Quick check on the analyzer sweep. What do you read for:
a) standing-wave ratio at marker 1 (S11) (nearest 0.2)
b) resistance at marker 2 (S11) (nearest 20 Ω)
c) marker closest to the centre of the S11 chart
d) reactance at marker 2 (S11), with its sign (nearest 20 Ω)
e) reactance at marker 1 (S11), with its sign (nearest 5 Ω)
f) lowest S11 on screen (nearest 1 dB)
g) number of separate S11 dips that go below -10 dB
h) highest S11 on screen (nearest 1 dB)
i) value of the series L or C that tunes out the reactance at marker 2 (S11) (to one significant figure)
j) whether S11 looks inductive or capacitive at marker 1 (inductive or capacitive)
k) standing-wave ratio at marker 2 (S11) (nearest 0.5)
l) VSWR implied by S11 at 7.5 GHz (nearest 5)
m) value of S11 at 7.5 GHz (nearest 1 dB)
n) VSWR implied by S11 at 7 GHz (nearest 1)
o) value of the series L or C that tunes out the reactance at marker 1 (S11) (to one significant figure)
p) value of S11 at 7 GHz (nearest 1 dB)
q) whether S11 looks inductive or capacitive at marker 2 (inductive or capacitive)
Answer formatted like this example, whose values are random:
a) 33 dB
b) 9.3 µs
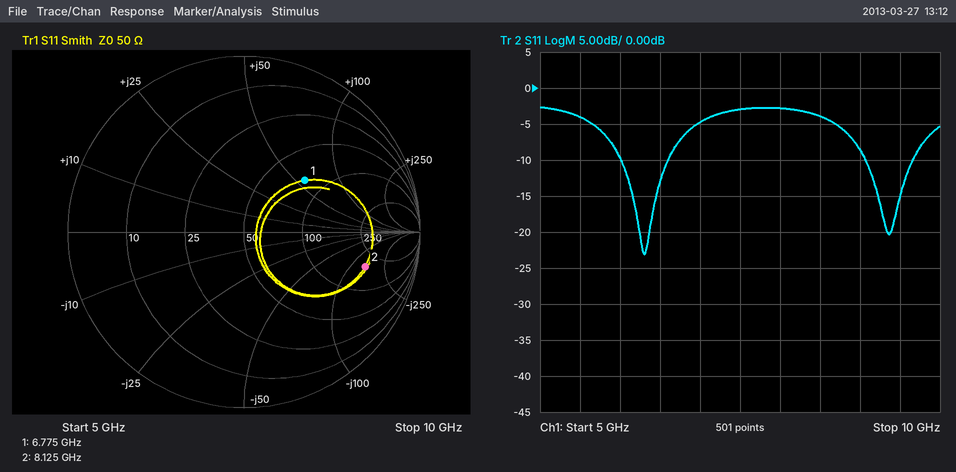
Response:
a) 2.6
b) 180 Ω
c) marker 1
d) -140 Ω
e) +55 Ω
f) -23 dB
g) 2
h) -3 dB
i) 3 nH
j) inductive
k) 6.0
l) 5
m) -3 dB
n) 4
o) 400 fF
p) -5 dB
q) capacitive
